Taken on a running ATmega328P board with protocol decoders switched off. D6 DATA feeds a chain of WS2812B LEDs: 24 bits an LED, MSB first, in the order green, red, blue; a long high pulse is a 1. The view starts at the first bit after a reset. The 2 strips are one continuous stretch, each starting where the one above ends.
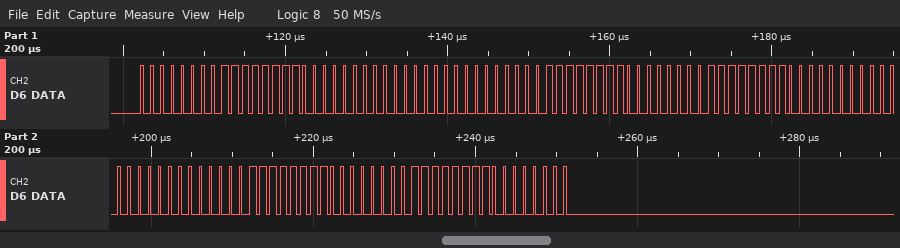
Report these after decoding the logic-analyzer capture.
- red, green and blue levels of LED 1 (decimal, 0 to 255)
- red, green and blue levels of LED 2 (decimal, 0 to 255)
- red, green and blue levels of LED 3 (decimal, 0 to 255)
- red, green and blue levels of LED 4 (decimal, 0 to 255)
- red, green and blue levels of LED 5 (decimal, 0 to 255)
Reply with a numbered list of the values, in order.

1. 255, 0, 0
2. 0, 0, 255
3. 255, 0, 0
4. 0, 0, 255
5. 255, 0, 0
